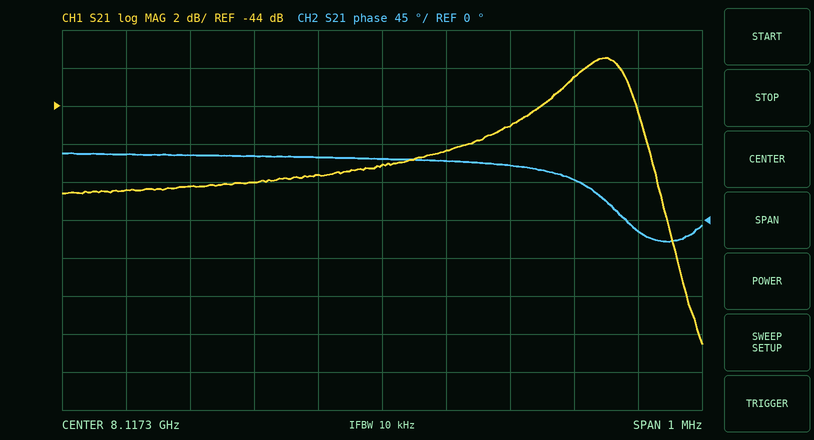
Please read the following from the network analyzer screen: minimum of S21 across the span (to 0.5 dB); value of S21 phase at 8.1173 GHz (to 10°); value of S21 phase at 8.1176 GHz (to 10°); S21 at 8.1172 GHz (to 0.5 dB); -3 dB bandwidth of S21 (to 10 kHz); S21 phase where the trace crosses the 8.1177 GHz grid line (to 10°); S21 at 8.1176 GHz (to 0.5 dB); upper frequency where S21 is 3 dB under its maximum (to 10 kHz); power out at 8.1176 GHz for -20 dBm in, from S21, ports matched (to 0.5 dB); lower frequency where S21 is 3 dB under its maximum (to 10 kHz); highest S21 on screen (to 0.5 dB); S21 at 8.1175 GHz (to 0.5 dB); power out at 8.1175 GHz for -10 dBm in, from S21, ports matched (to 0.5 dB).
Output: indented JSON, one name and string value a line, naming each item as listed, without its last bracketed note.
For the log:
{
  "minimum of S21 across the span": "-56.5 dB",
  "value of S21 phase at 8.1173 GHz": "70°",
  "value of S21 phase at 8.1176 GHz": "50°",
  "S21 at 8.1172 GHz": "-47.5 dB",
  "-3 dB bandwidth of S21": "170 kHz",
  "S21 phase where the trace crosses the 8.1177 GHz grid line": "-10°",
  "S21 at 8.1176 GHz": "-42.5 dB",
  "upper frequency where S21 is 3 dB under its maximum": "8.11770 GHz",
  "power out at 8.1176 GHz for -20 dBm in, from S21, ports matched": "-62.5 dBm",
  "lower frequency where S21 is 3 dB under its maximum": "8.11753 GHz",
  "highest S21 on screen": "-41.5 dB",
  "S21 at 8.1175 GHz": "-45.0 dB",
  "power out at 8.1175 GHz for -10 dBm in, from S21, ports matched": "-55.0 dBm"
}
